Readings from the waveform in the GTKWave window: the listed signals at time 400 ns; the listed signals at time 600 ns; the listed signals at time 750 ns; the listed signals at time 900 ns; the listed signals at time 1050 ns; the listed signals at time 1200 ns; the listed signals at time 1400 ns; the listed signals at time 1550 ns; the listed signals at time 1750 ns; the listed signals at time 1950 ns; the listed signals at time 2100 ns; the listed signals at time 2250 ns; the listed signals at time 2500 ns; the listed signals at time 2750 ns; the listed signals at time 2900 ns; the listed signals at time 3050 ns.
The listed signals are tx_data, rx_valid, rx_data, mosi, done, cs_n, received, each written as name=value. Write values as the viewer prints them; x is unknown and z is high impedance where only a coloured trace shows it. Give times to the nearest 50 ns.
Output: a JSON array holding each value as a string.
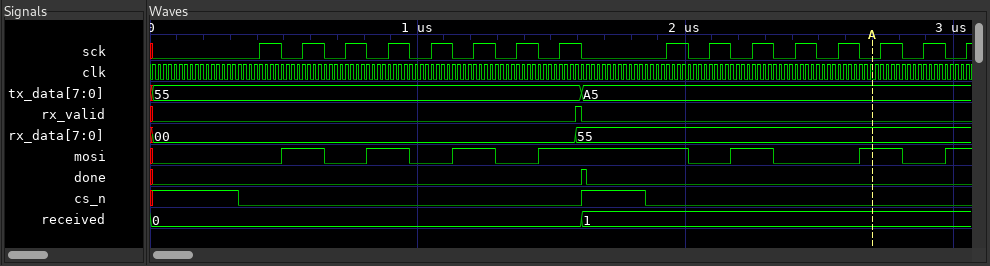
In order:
["tx_data=55, rx_valid=0, rx_data=00, mosi=0, done=0, cs_n=0, received=0", "tx_data=55, rx_valid=0, rx_data=00, mosi=1, done=0, cs_n=0, received=0", "tx_data=55, rx_valid=0, rx_data=00, mosi=0, done=0, cs_n=0, received=0", "tx_data=55, rx_valid=0, rx_data=00, mosi=1, done=0, cs_n=0, received=0", "tx_data=55, rx_valid=0, rx_data=00, mosi=0, done=0, cs_n=0, received=0", "tx_data=55, rx_valid=0, rx_data=00, mosi=1, done=0, cs_n=0, received=0", "tx_data=55, rx_valid=0, rx_data=00, mosi=0, done=0, cs_n=0, received=0", "tx_data=55, rx_valid=0, rx_data=00, mosi=1, done=0, cs_n=0, received=0", "tx_data=A5, rx_valid=0, rx_data=55, mosi=1, done=0, cs_n=1, received=1", "tx_data=A5, rx_valid=0, rx_data=55, mosi=1, done=0, cs_n=0, received=1", "tx_data=A5, rx_valid=0, rx_data=55, mosi=0, done=0, cs_n=0, received=1", "tx_data=A5, rx_valid=0, rx_data=55, mosi=1, done=0, cs_n=0, received=1", "tx_data=A5, rx_valid=0, rx_data=55, mosi=0, done=0, cs_n=0, received=1", "tx_data=A5, rx_valid=0, rx_data=55, mosi=1, done=0, cs_n=0, received=1", "tx_data=A5, rx_valid=0, rx_data=55, mosi=0, done=0, cs_n=0, received=1", "tx_data=A5, rx_valid=0, rx_data=55, mosi=1, done=0, cs_n=0, received=1"]
